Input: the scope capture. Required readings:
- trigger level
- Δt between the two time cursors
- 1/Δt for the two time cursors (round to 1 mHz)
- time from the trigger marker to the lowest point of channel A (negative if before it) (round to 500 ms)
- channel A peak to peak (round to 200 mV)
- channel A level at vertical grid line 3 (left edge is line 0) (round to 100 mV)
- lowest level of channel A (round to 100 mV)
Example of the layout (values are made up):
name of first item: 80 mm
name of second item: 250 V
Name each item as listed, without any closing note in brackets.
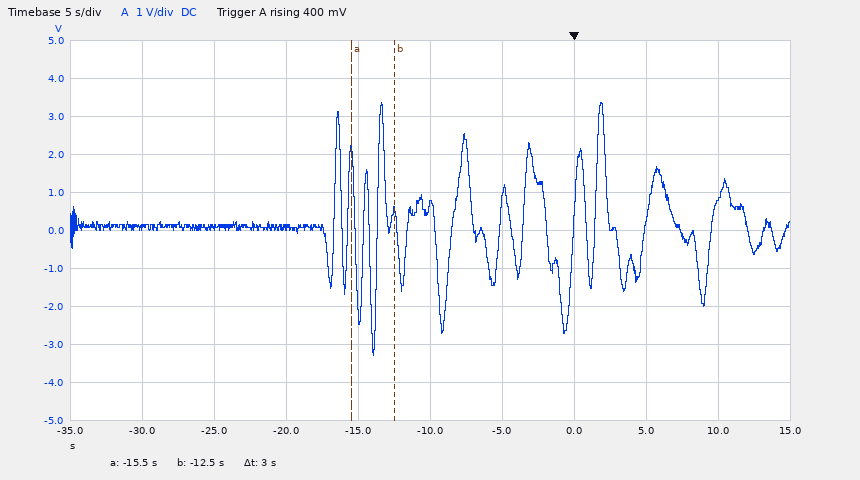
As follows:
trigger level: 400 mV
Δt between the two time cursors: 3 s
1/Δt for the two time cursors: 333 mHz
time from the trigger marker to the lowest point of channel A (negative if before it): -14.0 s
channel A peak to peak: 6.6 V
channel A level at vertical grid line 3 (left edge is line 0): 100 mV
lowest level of channel A: -3.3 V
